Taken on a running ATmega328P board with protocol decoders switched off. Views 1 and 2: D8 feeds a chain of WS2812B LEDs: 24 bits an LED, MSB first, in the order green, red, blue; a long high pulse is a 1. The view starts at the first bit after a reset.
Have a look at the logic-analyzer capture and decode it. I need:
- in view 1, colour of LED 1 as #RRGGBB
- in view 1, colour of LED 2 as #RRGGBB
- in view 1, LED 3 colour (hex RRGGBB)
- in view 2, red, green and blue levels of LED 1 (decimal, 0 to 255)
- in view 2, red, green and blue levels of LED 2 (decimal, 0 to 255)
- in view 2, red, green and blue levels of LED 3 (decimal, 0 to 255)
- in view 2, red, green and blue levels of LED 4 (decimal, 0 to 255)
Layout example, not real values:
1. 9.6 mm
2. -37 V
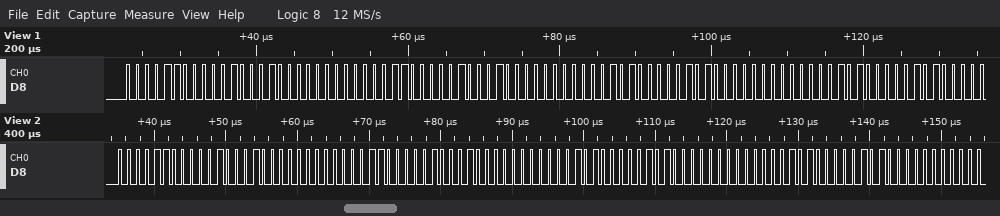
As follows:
1. #110C00
2. #110C00
3. #141400
4. 17, 12, 0
5. 17, 12, 0
6. 20, 20, 0
7. 20, 20, 0
